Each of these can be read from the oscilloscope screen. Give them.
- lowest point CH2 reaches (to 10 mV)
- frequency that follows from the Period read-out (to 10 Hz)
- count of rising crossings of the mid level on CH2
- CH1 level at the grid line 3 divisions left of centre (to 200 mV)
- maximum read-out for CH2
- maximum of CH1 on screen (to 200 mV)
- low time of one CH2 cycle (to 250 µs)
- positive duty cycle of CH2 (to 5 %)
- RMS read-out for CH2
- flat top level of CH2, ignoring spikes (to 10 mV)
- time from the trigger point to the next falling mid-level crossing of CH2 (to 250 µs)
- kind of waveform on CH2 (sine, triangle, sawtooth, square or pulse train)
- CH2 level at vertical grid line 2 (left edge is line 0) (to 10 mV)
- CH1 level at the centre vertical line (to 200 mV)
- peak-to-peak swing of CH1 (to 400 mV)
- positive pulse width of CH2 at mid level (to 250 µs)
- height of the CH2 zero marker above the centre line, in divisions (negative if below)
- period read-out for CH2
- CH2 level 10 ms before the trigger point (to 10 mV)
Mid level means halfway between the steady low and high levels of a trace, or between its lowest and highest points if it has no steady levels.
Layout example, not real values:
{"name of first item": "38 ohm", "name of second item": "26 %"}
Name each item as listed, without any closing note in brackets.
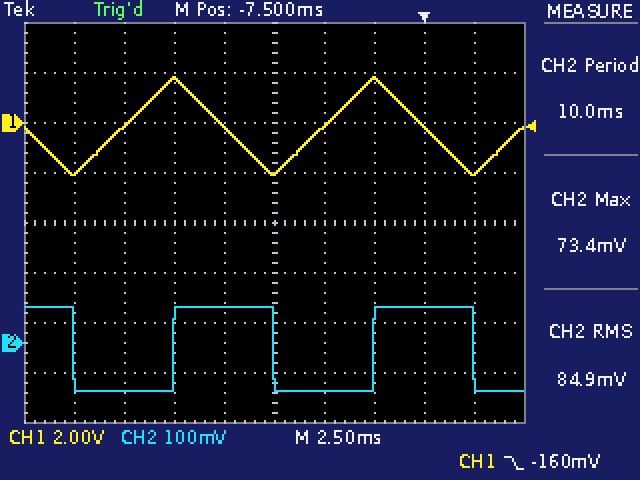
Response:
{"lowest point CH2 reaches": "-100 mV", "frequency that follows from the Period read-out": "100 Hz", "count of rising crossings of the mid level on CH2": "2", "CH1 level at the grid line 3 divisions left of centre": "-200 mV", "maximum read-out for CH2": "73.4 mV", "maximum of CH1 on screen": "1.8 V", "low time of one CH2 cycle": "5.00 ms", "positive duty cycle of CH2": "50 %", "RMS read-out for CH2": "84.9 mV", "flat top level of CH2, ignoring spikes": "70 mV", "time from the trigger point to the next falling mid-level crossing of CH2": "2.50 ms", "kind of waveform on CH2": "square", "CH2 level at vertical grid line 2 (left edge is line 0)": "-100 mV", "CH1 level at the centre vertical line": "-2.0 V", "peak-to-peak swing of CH1": "4.0 V", "positive pulse width of CH2 at mid level": "5.00 ms", "height of the CH2 zero marker above the centre line, in divisions": "-2.4 div", "period read-out for CH2": "10.0 ms", "CH2 level 10 ms before the trigger point": "70 mV"}
